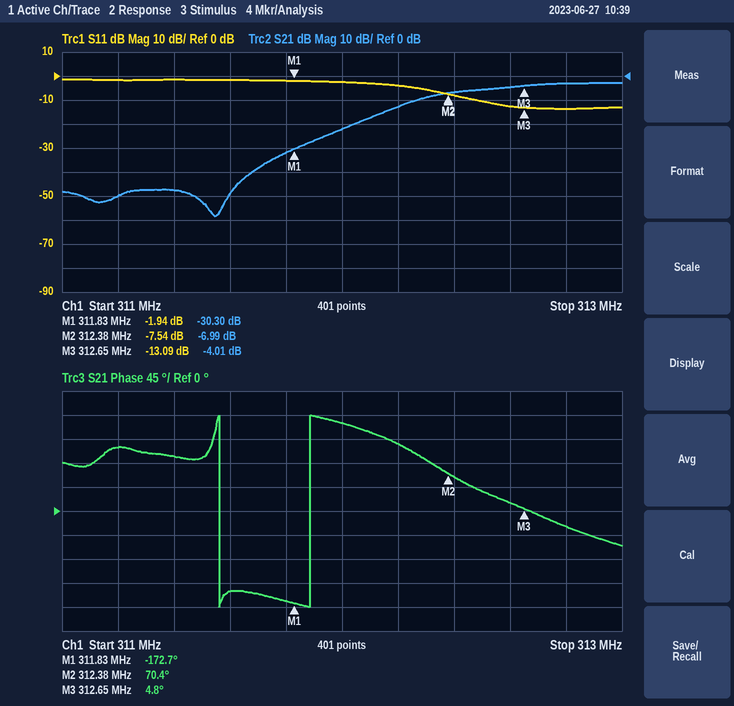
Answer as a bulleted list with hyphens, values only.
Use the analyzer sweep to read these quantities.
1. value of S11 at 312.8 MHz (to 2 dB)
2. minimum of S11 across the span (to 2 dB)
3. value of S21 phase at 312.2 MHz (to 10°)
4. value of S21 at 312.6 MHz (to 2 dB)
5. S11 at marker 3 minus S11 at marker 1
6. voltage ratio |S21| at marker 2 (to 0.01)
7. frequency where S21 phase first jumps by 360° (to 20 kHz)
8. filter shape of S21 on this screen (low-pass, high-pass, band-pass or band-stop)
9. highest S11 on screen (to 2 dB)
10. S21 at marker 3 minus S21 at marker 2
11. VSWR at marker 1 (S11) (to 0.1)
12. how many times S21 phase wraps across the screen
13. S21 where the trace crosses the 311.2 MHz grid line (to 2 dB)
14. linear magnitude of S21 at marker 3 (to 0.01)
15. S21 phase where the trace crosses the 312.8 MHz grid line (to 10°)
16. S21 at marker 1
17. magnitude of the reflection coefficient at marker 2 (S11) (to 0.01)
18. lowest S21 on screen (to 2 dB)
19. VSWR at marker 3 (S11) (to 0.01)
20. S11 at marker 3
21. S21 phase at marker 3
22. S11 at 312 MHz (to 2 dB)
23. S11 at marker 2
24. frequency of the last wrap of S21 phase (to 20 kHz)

- -14 dB
- -14 dB
- 130°
- -4 dB
- -11.15 dB
- 0.45
- 311.56 MHz
- high-pass
- -2 dB
- 2.98 dB
- 9.0
- 2
- -50 dB
- 0.63
- -30°
- -30.30 dB
- 0.42
- -58 dB
- 1.57
- -13.09 dB
- 4.8°
- -2 dB
- -7.54 dB
- 311.88 MHz
